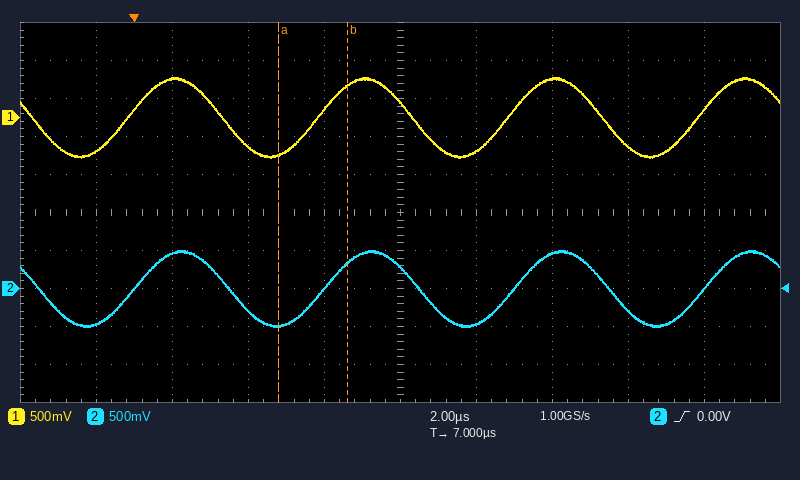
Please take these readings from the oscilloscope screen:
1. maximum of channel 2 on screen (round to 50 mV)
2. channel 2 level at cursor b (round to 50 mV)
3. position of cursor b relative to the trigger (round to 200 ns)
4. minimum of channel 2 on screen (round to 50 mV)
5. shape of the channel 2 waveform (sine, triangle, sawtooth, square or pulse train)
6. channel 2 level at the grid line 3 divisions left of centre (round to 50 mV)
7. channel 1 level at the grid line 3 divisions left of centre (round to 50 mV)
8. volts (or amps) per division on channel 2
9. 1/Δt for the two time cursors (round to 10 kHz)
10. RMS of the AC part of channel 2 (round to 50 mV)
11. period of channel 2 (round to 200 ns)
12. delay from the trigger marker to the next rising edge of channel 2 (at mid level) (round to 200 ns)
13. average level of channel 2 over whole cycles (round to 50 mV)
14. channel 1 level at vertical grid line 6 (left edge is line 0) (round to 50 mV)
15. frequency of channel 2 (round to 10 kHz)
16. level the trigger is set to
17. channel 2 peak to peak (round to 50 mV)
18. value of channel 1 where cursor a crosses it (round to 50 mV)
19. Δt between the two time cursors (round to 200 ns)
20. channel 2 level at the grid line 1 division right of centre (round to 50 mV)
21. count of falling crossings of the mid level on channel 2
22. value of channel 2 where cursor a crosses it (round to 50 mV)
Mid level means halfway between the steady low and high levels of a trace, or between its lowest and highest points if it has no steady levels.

500 mV
350 mV
+5.6 µs
-500 mV
sine
450 mV
500 mV
500 mV
560 kHz
350 mV
5.0 µs
5.0 µs
0 mV
-450 mV
200 kHz
0.00 V
1.00 V
-500 mV
1.8 µs
-450 mV
4
-500 mV
